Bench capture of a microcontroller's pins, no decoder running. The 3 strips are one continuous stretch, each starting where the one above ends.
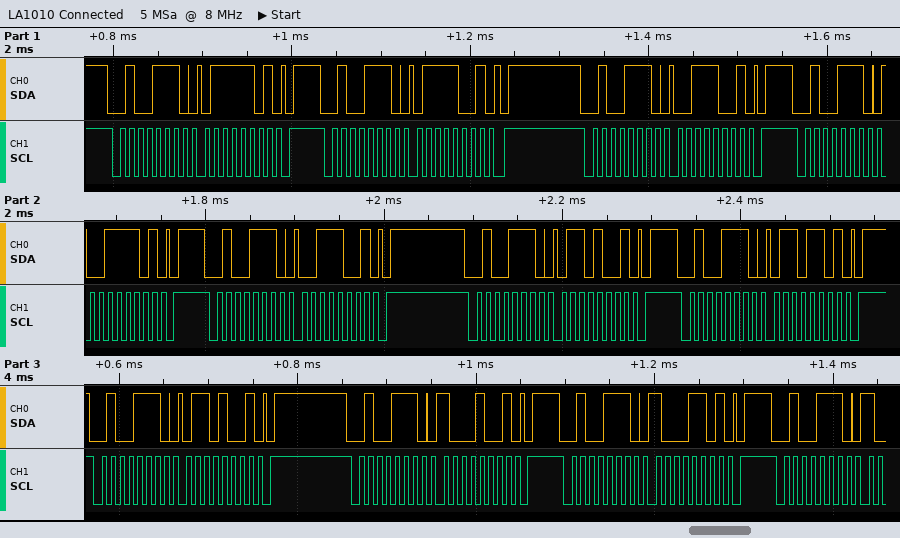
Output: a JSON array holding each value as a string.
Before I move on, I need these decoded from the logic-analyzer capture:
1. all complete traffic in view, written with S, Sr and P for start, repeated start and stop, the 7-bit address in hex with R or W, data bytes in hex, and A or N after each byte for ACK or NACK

["S 27W A 7D A P S 27W A 79 A P S 27W A 39 A P S 27W A 3D A P S 27W A 39 A P S 27W A 69 A P S 27W A 6D A P S 27W A 69 A P S 27W A 89 A P S 27W A 8D A P S 27W A"]
